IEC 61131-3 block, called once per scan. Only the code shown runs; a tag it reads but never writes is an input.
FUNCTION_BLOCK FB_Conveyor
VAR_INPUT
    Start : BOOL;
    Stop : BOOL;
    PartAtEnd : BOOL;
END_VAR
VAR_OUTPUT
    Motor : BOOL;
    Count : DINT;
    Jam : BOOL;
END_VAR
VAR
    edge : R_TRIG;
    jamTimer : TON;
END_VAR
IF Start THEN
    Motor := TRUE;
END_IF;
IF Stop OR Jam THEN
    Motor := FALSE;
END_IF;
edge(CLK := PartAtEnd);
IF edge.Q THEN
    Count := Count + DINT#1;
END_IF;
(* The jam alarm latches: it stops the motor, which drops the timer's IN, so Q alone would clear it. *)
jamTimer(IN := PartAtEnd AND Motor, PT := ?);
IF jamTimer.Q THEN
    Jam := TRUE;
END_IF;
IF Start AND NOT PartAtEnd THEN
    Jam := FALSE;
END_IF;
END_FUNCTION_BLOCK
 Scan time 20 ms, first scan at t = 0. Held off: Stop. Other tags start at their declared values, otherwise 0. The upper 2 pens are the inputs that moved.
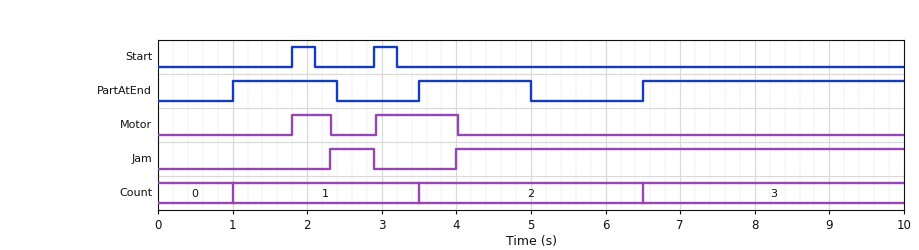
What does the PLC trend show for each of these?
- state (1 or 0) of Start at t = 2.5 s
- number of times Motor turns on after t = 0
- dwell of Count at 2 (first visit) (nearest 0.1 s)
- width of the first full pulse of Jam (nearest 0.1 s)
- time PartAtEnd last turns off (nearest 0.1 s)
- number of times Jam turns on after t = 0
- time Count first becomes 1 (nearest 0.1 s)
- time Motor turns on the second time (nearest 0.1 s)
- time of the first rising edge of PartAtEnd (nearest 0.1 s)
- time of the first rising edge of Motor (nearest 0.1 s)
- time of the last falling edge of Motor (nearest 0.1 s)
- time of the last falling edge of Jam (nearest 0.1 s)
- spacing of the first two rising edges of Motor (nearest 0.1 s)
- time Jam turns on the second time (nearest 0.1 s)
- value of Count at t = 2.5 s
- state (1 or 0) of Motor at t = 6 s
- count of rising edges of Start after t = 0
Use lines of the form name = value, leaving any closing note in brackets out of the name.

state (1 or 0) of Start at t = 2.5 s = 0
number of times Motor turns on after t = 0 = 2
dwell of Count at 2 (first visit) = 3.0 s
width of the first full pulse of Jam = 0.6 s
time PartAtEnd last turns off = 5.0 s
number of times Jam turns on after t = 0 = 2
time Count first becomes 1 = 1.0 s
time Motor turns on the second time = 2.9 s
time of the first rising edge of PartAtEnd = 1.0 s
time of the first rising edge of Motor = 1.8 s
time of the last falling edge of Motor = 4.0 s
time of the last falling edge of Jam = 2.9 s
spacing of the first two rising edges of Motor = 1.1 s
time Jam turns on the second time = 4.0 s
value of Count at t = 2.5 s = 1
state (1 or 0) of Motor at t = 6 s = 0
count of rising edges of Start after t = 0 = 2
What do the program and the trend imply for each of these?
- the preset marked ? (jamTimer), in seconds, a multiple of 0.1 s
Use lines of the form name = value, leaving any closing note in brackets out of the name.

the preset marked ? (jamTimer), in seconds, a multiple of 0.1 s = 0.5 s
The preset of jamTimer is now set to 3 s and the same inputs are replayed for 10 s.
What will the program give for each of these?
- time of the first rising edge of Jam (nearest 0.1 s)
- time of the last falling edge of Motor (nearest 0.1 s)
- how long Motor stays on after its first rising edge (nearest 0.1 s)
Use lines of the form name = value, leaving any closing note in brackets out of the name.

time of the first rising edge of Jam = 9.5 s
time of the last falling edge of Motor = 9.5 s
how long Motor stays on after its first rising edge = 7.7 s
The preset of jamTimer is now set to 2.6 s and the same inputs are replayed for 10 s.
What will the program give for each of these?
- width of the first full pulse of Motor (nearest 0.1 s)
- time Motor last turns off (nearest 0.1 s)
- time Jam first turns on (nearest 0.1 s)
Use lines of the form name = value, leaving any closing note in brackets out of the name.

width of the first full pulse of Motor = 7.3 s
time Motor last turns off = 9.1 s
time Jam first turns on = 9.1 s
